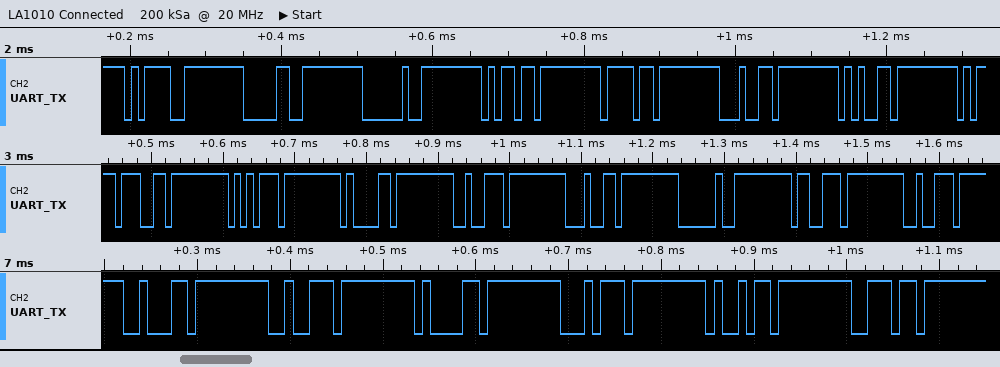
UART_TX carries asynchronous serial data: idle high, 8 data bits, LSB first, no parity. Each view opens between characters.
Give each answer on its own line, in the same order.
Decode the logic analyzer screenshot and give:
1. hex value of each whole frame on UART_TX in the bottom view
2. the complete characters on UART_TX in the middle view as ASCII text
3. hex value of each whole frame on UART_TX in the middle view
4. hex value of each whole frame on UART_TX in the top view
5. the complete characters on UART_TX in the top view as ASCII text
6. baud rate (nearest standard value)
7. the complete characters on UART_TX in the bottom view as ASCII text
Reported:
62, 72, 61, 74, 69, 6E
"guard sr"
67, 75, 61, 72, 64, 20, 73, 72
3D, 30, 20, 6D, 6F, 64, 65
"=0 mode"
115200 baud
"bratin"
